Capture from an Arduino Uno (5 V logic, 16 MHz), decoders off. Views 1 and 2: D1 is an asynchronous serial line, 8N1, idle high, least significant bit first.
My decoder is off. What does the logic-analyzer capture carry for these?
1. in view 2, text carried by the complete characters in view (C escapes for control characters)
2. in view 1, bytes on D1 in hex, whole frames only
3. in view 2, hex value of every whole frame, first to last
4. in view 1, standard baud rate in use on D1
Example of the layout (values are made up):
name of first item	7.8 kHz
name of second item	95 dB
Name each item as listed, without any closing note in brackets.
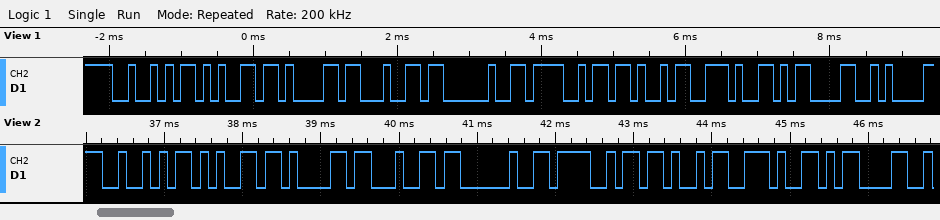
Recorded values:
in view 2, text carried by the complete characters in view	"Read OK.\r"
in view 1, bytes on D1 in hex, whole frames only	0x52 0x65 0x61 0x64 0x20 0x4F 0x4B 0x2E 0x0D 0x0A
in view 2, hex value of every whole frame, first to last	52 65 61 64 20 4F 4B 2E 0D
in view 1, standard baud rate in use on D1	9600 baud
